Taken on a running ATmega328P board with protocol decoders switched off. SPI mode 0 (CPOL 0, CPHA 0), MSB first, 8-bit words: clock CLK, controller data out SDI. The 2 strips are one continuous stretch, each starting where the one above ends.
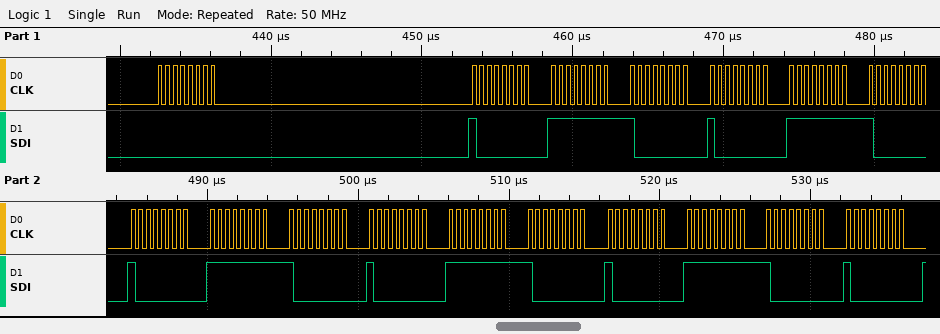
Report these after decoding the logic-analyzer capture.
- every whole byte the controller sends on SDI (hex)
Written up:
00 80 FF 80 80 FF 80 80 FF 80 80 FF 80 80 FF 80 80
